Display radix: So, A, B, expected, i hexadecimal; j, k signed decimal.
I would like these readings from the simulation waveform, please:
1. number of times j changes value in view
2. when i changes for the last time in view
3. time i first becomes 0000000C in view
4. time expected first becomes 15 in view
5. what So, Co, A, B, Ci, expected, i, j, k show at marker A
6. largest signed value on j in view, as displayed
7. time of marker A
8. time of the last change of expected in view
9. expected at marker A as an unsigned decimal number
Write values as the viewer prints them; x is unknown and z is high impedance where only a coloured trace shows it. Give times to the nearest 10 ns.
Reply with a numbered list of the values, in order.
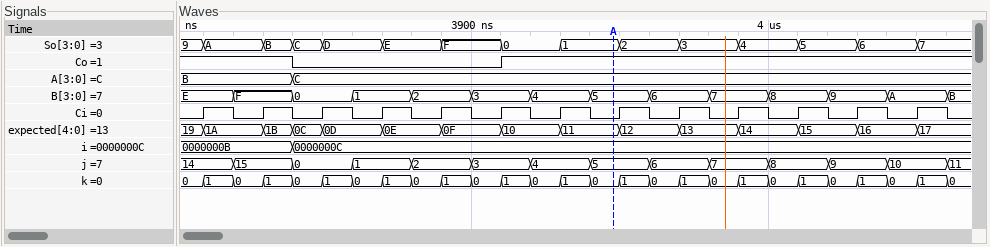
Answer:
1. 13
2. 3840 ns
3. 3840 ns
4. 4010 ns
5. So=1, Co=1, A=C, B=5, Ci=0, expected=11, i=0000000C, j=5, k=0
6. 15
7. 3950 ns
8. 4050 ns
9. 17
